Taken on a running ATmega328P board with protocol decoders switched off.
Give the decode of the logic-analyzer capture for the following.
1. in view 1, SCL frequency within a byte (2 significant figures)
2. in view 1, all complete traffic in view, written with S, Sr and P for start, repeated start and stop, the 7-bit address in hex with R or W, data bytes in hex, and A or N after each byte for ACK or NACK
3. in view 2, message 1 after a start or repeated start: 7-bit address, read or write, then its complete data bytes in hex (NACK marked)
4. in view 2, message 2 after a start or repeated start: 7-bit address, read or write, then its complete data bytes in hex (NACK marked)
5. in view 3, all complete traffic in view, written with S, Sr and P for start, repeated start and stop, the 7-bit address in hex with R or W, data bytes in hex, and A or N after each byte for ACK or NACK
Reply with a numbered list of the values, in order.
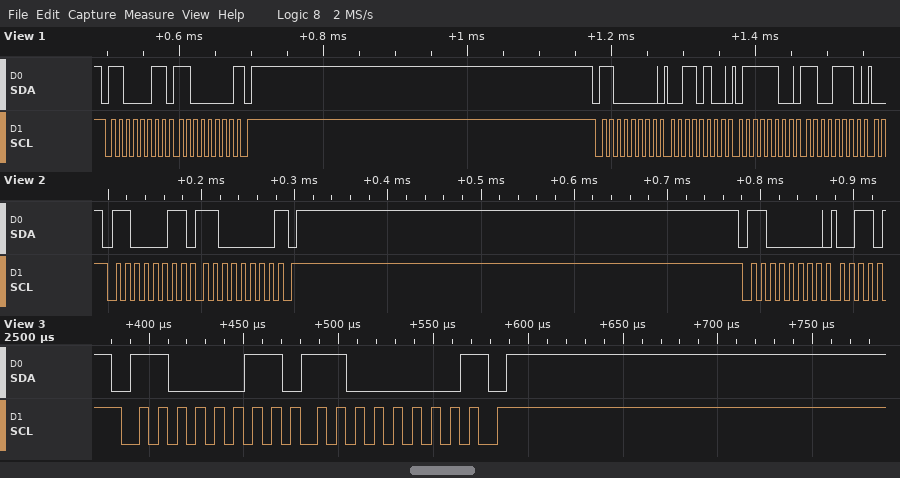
1. 100 kHz
2. S 61R A C0 N P S 60W A 34 A 7C A CE A
3. 0x61 read: C0 NACK
4. 0x60 write
5. S 61R A C0 N P
